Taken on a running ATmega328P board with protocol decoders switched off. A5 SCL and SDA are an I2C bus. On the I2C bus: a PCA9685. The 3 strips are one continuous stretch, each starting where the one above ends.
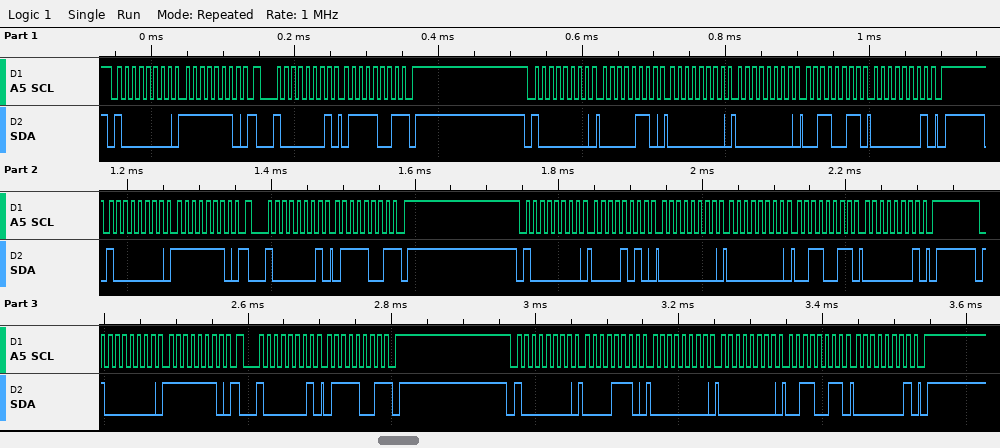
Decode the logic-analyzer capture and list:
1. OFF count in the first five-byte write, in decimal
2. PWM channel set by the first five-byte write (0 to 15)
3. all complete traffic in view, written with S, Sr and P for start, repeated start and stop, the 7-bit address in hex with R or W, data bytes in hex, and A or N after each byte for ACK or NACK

307
0
S 40W A FE A Sr 40R A 79 N P S 40W A 06 A 00 A 00 A 33 A 01 A P S 40W A FE A Sr 40R A 79 N P S 40W A 0A A 00 A 00 A 33 A 01 A P S 40W A FE A Sr 40R A 79 N P S 40W A 0E A 00 A 00 A 33 A 01 A P
